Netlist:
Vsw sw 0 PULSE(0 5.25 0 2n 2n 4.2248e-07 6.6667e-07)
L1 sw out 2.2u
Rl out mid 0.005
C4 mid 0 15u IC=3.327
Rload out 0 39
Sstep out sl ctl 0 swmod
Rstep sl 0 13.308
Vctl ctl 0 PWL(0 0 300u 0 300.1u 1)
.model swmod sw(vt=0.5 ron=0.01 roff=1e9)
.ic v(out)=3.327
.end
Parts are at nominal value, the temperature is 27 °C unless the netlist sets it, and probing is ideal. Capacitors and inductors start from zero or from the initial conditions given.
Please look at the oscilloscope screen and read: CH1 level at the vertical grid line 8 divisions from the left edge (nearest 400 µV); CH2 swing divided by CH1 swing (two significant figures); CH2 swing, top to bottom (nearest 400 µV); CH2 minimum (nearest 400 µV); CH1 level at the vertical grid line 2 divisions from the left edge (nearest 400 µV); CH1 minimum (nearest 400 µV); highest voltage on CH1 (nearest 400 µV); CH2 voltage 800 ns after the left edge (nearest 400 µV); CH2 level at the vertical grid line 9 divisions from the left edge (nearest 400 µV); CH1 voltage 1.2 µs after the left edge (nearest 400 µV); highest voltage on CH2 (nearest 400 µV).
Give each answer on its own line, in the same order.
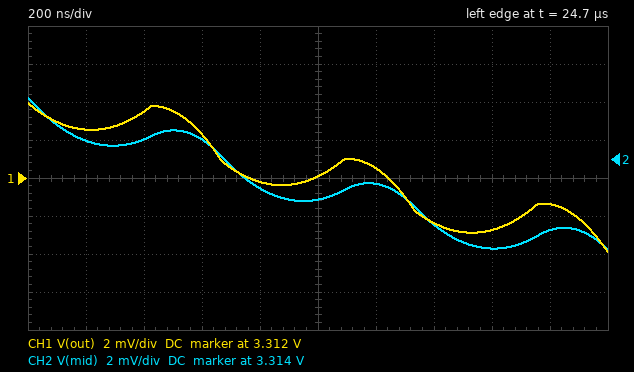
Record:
3.3092 V
1.0
8.0 mV
3.3092 V
3.3156 V
3.3080 V
3.3160 V
3.3124 V
3.3104 V
3.3124 V
3.3172 V
